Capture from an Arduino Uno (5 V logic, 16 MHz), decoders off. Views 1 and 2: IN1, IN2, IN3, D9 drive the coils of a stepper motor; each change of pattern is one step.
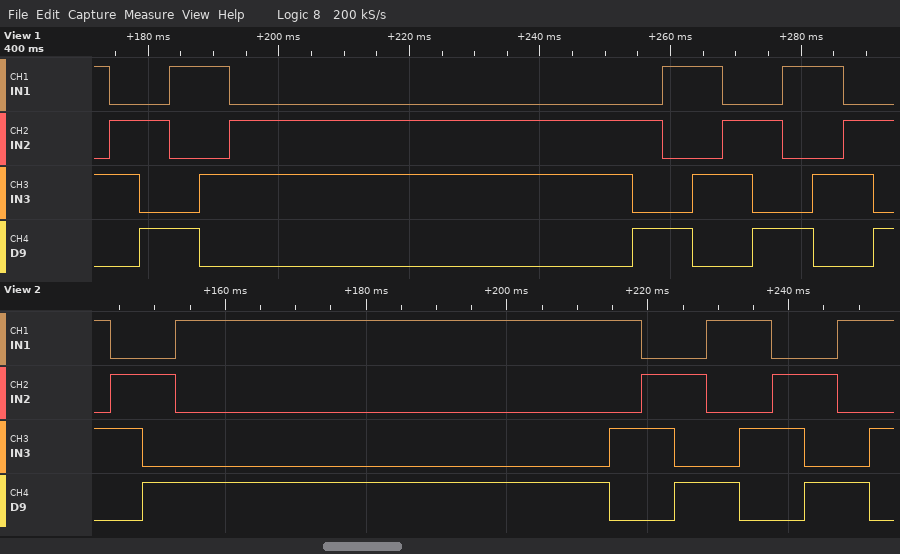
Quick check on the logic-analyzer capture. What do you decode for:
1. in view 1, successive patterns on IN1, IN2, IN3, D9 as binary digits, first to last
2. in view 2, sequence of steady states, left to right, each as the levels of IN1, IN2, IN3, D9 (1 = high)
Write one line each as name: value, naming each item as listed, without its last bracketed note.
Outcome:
in view 1, successive patterns on IN1, IN2, IN3, D9 as binary digits, first to last: 1010 0110 0101 1001 1010 0110 0101 1001 1010 0110 0101 1001 1010 0110 0101
in view 2, sequence of steady states, left to right, each as the levels of IN1, IN2, IN3, D9: 1010 0110 0101 1001 1010 0110 0101 1001 1010 0110 0101 1001 1010
